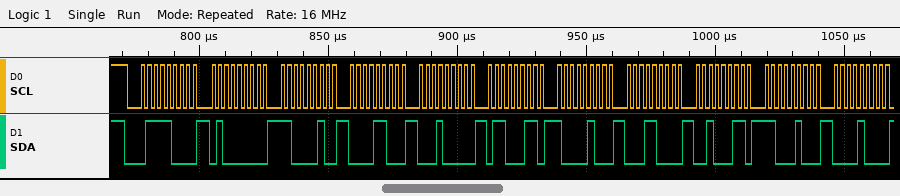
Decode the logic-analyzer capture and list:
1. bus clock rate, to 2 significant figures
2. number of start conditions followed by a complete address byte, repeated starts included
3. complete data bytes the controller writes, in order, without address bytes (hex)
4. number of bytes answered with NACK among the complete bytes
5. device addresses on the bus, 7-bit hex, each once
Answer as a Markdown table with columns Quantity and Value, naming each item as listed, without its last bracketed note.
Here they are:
| Quantity | Value |
|---|---|
| bus clock rate, to 2 significant figures | 400 kHz |
| number of start conditions followed by a complete address byte, repeated starts included | 1 |
| complete data bytes the controller writes, in order, without address bytes | 40 C2 0C 10 63 84 18 23 C4 08 |
| number of bytes answered with NACK among the complete bytes | 0 |
| device addresses on the bus, 7-bit hex, each once | 0x3C |
